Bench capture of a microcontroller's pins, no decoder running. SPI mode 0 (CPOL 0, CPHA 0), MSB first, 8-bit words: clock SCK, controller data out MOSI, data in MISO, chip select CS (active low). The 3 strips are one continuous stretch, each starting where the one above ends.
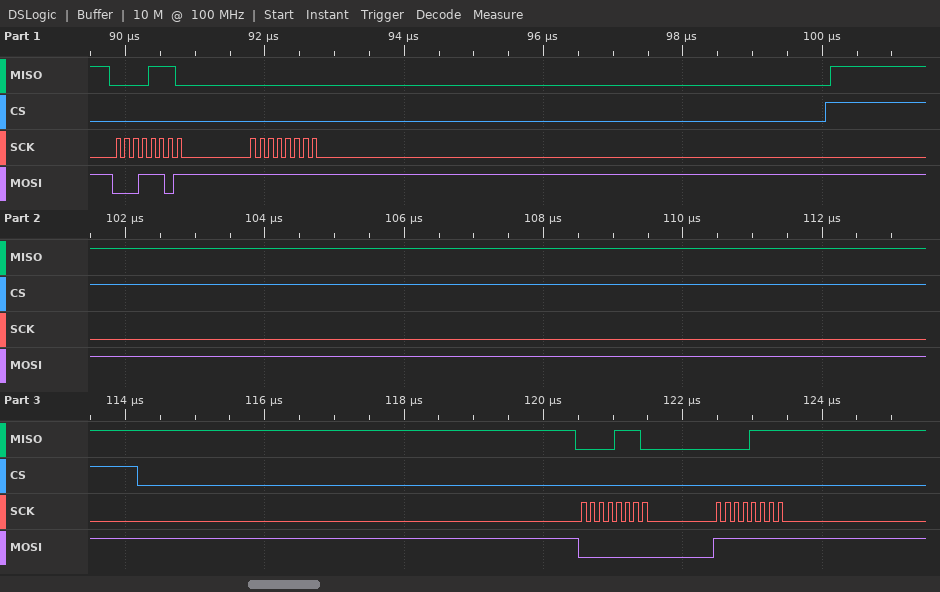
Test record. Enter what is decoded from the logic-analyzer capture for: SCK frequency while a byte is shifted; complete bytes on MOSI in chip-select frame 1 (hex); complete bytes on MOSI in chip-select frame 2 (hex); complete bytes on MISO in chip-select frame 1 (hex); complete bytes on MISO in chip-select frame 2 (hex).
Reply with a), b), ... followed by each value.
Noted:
a) 8 MHz
b) 1D FF
c) 00 FF
d) 0E 00
e) 0E 0F
